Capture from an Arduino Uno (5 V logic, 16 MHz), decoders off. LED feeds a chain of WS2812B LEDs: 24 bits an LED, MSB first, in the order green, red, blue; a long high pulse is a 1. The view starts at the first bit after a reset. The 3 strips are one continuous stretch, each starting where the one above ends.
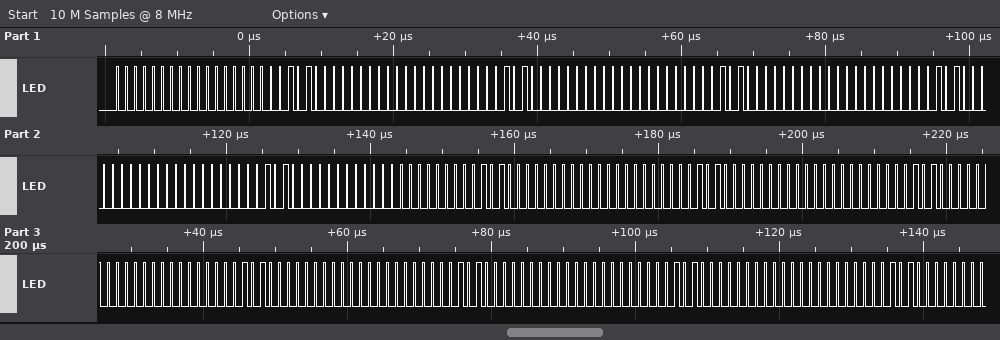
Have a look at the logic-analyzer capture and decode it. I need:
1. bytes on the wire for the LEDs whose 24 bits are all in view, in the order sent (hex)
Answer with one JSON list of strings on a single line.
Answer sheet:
["00 00 14 00 00 14 00 00 14 00 00 14 00 00 14 00 00 14 00 00 14 00 00 14 00 00 14 00 00 14 00 00 14 00 00 14"]
